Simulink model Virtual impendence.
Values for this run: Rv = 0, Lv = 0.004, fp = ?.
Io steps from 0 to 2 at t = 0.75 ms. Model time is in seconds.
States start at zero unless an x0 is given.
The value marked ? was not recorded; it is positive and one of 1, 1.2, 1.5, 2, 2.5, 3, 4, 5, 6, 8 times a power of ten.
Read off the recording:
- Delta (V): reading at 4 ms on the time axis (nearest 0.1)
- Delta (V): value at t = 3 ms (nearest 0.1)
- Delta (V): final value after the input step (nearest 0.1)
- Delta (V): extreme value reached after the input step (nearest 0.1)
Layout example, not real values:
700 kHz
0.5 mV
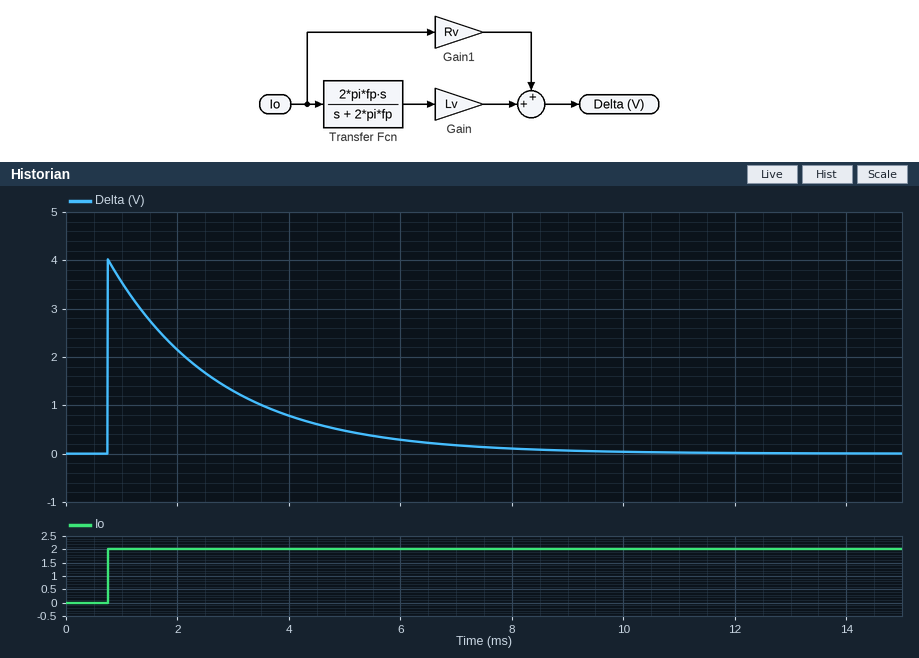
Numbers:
0.8
1.3
0.0
4.0
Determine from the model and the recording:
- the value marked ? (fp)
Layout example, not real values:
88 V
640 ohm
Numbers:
80
